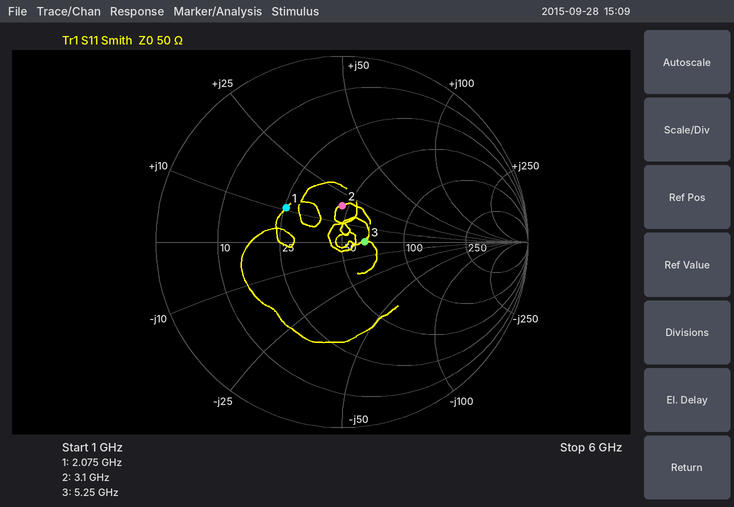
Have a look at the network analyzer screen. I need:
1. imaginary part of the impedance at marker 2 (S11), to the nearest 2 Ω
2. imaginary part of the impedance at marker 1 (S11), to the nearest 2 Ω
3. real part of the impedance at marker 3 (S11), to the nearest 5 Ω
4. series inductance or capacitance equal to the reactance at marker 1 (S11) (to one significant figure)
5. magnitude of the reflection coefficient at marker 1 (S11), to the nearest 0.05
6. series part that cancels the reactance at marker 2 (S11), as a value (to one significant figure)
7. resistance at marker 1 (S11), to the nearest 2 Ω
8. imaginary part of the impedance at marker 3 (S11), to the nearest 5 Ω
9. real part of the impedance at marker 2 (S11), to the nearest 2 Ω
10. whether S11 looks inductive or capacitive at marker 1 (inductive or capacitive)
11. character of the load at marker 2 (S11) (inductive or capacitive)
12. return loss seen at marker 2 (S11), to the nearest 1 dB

+18 Ω
+10 Ω
65 Ω
800 pH
0.35
3 pF
26 Ω
0 Ω
46 Ω
inductive
inductive
14 dB
